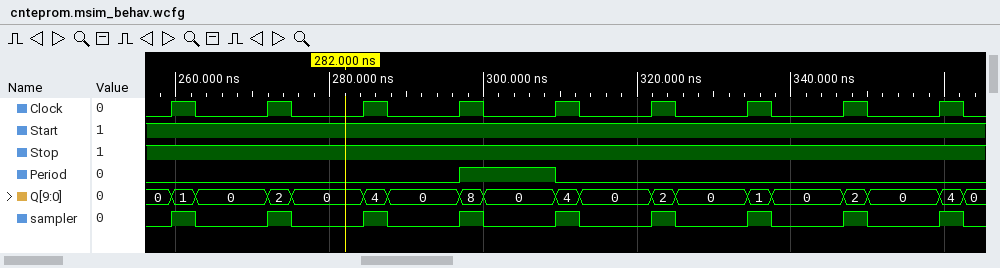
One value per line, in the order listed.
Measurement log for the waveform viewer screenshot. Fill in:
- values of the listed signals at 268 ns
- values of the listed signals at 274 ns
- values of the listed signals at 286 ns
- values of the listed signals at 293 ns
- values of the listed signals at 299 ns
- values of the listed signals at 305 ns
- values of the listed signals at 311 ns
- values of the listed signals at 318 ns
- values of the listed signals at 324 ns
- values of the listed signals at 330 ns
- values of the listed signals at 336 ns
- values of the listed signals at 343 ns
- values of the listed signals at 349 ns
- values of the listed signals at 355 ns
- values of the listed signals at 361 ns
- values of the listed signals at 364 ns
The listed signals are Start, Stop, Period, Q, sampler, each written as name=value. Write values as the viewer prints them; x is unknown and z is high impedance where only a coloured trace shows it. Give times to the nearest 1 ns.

Start=1, Stop=1, Period=0, Q=0, sampler=0
Start=1, Stop=1, Period=0, Q=2, sampler=1
Start=1, Stop=1, Period=0, Q=4, sampler=1
Start=1, Stop=1, Period=0, Q=0, sampler=0
Start=1, Stop=1, Period=1, Q=8, sampler=1
Start=1, Stop=1, Period=1, Q=0, sampler=0
Start=1, Stop=1, Period=0, Q=4, sampler=1
Start=1, Stop=1, Period=0, Q=0, sampler=0
Start=1, Stop=1, Period=0, Q=2, sampler=1
Start=1, Stop=1, Period=0, Q=0, sampler=0
Start=1, Stop=1, Period=0, Q=1, sampler=1
Start=1, Stop=1, Period=0, Q=0, sampler=0
Start=1, Stop=1, Period=0, Q=2, sampler=1
Start=1, Stop=1, Period=0, Q=0, sampler=0
Start=1, Stop=1, Period=0, Q=4, sampler=1
Start=1, Stop=1, Period=0, Q=0, sampler=0
